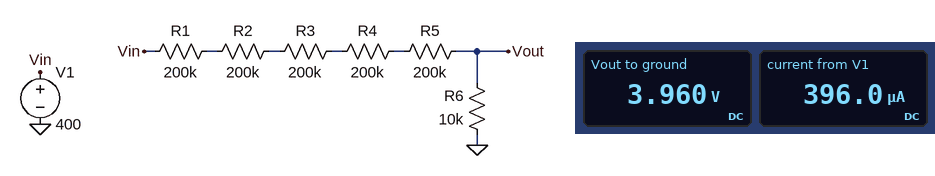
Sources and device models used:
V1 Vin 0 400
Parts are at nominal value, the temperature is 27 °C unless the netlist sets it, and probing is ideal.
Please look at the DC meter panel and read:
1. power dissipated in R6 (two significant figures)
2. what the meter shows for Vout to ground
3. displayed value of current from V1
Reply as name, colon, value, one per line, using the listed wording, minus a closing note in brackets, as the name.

power dissipated in R6: 1.6 mW
what the meter shows for Vout to ground: 3.960 V
displayed value of current from V1: 396.0 µA
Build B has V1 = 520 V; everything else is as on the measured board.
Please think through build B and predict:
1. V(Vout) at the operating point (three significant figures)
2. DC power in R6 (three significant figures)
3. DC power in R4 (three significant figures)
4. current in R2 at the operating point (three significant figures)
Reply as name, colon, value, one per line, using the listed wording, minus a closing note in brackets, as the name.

V(Vout) at the operating point: 5.15 V
DC power in R6: 2.65 mW
DC power in R4: 53.0 mW
current in R2 at the operating point: 515 µA
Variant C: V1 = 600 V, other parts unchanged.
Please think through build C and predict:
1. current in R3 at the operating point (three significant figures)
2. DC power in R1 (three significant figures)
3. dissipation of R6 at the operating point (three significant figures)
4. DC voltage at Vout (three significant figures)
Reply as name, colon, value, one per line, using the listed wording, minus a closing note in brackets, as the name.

current in R3 at the operating point: 594 µA
DC power in R1: 70.6 mW
dissipation of R6 at the operating point: 3.53 mW
DC voltage at Vout: 5.94 V
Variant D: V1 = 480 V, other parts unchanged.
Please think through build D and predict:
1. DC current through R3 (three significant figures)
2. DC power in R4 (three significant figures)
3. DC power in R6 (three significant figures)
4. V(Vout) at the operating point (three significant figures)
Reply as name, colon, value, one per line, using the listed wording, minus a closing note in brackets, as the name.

DC current through R3: 475 µA
DC power in R4: 45.2 mW
DC power in R6: 2.26 mW
V(Vout) at the operating point: 4.75 V
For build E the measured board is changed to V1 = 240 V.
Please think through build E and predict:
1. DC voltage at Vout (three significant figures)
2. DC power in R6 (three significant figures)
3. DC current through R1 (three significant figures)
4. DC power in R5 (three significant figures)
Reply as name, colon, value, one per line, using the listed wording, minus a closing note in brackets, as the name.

DC voltage at Vout: 2.38 V
DC power in R6: 565 µW
DC current through R1: 238 µA
DC power in R5: 11.3 mW
